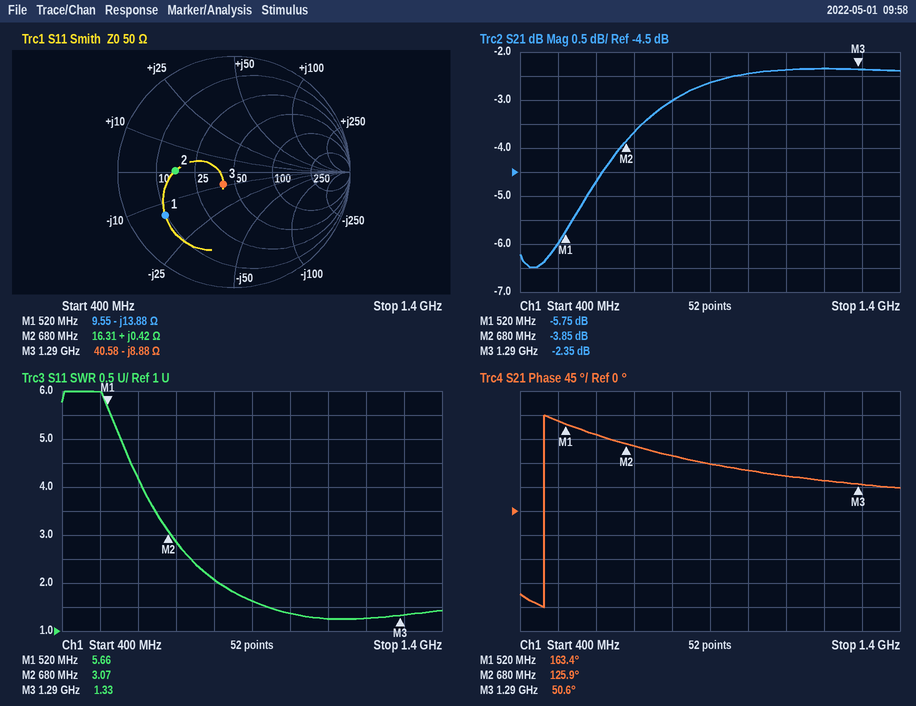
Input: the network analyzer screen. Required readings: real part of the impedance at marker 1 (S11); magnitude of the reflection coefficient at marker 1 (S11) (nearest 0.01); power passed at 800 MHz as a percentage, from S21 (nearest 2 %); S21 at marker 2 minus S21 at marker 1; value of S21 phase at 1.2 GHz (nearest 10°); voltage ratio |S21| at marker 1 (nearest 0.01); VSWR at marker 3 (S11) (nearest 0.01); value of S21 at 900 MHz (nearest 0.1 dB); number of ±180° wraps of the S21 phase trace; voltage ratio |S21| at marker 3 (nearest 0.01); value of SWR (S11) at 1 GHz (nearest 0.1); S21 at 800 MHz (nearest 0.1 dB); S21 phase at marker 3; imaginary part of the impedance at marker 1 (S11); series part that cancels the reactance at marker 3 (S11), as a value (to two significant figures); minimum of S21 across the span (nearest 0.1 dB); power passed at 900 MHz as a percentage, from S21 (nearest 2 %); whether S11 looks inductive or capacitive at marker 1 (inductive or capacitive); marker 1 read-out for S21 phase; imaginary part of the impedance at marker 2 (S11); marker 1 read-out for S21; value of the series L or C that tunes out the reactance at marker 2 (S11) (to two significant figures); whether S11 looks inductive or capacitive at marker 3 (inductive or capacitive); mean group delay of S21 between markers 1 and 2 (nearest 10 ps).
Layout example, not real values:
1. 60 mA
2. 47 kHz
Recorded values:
1. 9.55 Ω
2. 0.70
3. 50 %
4. 1.90 dB
5. 60°
6. 0.52
7. 1.33
8. -2.6 dB
9. 1
10. 0.76
11. 1.4
12. -3.0 dB
13. 50.6°
14. -13.88 Ω
15. 1.1 nH
16. -6.5 dB
17. 54 %
18. capacitive
19. 163.4°
20. +0.42 Ω
21. -5.75 dB
22. 560 pF
23. capacitive
24. 650 ps
